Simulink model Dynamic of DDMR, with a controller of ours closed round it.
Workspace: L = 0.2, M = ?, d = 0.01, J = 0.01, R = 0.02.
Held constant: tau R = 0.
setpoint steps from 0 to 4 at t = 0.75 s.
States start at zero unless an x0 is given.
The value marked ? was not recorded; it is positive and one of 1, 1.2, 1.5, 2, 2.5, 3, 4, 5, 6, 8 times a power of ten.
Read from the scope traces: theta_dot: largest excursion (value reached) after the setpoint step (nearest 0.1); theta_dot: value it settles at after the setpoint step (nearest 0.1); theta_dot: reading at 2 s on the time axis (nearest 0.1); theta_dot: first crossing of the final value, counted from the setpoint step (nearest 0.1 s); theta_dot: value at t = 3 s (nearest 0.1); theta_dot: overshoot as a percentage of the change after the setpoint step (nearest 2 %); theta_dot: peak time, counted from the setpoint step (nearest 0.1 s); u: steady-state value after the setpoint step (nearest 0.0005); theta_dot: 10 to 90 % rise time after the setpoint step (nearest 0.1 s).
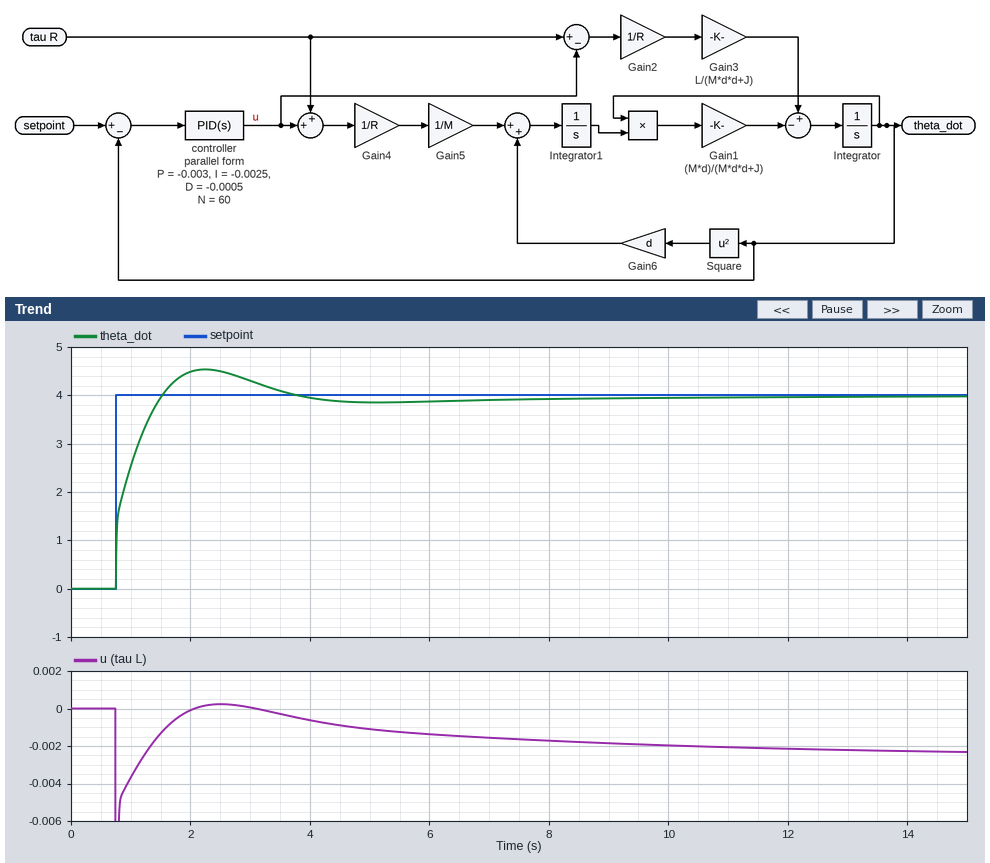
4.5
4.0
4.5
0.8 s
4.3
14 %
1.5 s
-0.0025
0.6 s
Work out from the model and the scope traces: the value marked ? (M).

0.8
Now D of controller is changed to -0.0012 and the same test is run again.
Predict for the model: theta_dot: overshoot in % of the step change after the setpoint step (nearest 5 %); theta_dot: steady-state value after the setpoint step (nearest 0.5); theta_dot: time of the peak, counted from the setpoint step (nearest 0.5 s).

10 %
4.0
2.0 s
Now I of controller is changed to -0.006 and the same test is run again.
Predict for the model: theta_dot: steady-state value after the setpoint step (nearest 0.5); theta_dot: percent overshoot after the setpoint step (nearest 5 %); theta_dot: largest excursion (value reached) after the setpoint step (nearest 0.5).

4.0
20 %
5.0
